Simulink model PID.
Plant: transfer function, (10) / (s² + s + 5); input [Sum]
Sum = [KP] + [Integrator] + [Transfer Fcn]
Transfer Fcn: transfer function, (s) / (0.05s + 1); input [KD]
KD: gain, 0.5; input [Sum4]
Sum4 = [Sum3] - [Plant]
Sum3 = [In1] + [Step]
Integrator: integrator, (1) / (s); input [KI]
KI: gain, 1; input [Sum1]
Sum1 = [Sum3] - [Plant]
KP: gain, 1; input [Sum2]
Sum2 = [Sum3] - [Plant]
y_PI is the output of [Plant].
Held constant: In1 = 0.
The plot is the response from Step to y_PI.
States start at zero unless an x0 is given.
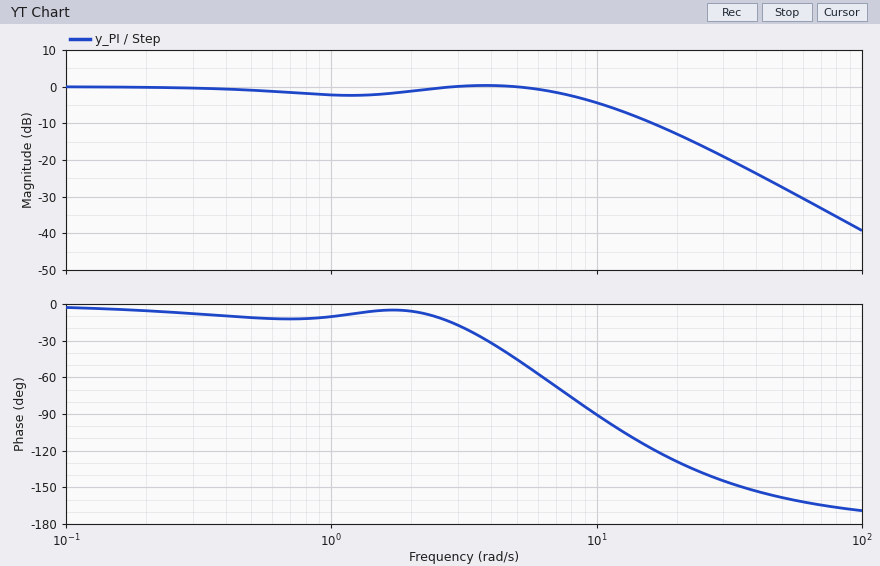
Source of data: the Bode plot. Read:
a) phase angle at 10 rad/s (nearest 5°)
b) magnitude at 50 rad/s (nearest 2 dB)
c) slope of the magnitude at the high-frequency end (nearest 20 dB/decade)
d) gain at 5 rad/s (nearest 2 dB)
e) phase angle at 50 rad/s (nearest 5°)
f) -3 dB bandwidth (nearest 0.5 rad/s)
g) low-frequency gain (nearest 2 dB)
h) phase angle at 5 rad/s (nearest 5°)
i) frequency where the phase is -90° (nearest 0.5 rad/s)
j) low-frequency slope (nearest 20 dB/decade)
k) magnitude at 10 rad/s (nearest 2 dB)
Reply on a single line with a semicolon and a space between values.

-90°; -28 dB; -40 dB/decade; 0 dB; -160°; 8.5 rad/s; 0 dB; -45°; 10.0 rad/s; 0 dB/decade; -4 dB
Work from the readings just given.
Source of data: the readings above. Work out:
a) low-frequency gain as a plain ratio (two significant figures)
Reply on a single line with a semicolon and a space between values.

1.0
